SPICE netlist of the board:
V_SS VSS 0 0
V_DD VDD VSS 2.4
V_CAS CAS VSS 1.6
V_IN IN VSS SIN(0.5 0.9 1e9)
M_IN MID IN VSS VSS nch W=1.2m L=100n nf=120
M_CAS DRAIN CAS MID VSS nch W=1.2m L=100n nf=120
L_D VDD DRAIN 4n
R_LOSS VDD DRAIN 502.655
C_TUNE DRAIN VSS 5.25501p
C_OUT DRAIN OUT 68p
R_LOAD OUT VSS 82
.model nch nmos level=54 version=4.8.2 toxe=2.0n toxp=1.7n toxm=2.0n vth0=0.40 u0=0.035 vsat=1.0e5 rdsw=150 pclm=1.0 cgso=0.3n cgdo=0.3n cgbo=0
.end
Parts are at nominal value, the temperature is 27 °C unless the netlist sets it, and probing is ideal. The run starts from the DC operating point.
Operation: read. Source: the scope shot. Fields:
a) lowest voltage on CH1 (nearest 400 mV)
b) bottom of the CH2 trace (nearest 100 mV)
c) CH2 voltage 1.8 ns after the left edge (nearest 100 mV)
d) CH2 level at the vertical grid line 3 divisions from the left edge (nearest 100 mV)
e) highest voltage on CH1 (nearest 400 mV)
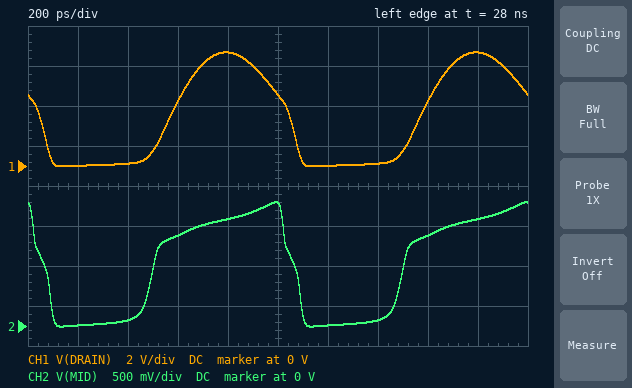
0 V
0 V
1.3 V
1.1 V
5.6 V
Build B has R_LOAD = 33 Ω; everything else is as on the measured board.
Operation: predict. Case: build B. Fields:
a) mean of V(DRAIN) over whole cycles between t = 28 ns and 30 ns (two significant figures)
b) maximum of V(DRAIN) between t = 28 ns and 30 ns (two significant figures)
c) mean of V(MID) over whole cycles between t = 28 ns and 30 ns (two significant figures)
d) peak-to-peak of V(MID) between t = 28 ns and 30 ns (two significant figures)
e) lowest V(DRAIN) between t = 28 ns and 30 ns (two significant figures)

2.4 V
5.2 V
800 mV
1.5 V
61 mV
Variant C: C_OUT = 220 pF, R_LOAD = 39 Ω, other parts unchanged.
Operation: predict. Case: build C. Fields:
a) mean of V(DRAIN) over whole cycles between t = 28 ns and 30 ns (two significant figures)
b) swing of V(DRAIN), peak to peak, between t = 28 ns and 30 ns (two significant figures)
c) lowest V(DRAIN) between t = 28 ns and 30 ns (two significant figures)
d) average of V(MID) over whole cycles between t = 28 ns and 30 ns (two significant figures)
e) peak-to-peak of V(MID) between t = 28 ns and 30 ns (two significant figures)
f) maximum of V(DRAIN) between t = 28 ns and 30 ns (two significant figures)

2.4 V
5.3 V
42 mV
790 mV
1.5 V
5.4 V
